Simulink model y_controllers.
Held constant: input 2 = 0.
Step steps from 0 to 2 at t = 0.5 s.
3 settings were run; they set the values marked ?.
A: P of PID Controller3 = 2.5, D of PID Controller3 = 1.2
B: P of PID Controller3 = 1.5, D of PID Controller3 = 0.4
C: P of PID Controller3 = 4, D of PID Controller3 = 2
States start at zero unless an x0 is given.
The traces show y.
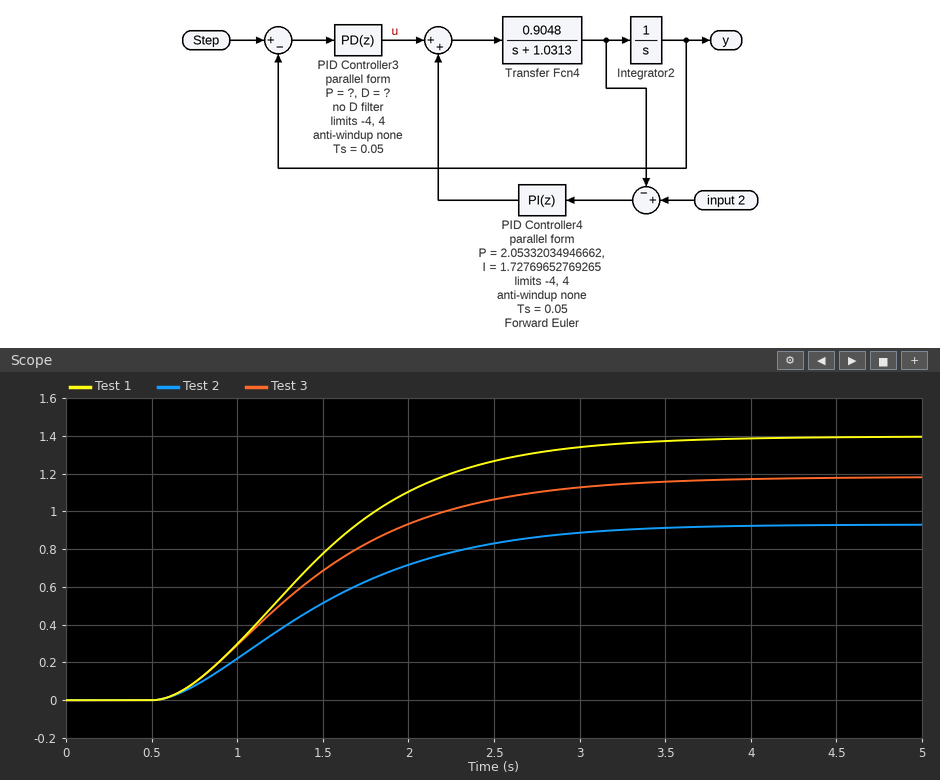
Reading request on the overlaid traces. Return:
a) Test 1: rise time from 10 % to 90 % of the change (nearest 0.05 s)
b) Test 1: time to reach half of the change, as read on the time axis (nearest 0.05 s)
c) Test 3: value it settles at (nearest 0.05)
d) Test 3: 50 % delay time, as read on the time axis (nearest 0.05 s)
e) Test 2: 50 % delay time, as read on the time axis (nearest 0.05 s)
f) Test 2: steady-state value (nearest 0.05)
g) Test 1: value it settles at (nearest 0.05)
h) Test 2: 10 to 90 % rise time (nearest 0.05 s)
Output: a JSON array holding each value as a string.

["1.65 s", "1.40 s", "1.20", "1.35 s", "1.40 s", "0.95", "1.40", "1.75 s"]
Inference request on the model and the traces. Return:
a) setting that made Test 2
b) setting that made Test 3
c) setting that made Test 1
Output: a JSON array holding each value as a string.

["B", "A", "C"]
